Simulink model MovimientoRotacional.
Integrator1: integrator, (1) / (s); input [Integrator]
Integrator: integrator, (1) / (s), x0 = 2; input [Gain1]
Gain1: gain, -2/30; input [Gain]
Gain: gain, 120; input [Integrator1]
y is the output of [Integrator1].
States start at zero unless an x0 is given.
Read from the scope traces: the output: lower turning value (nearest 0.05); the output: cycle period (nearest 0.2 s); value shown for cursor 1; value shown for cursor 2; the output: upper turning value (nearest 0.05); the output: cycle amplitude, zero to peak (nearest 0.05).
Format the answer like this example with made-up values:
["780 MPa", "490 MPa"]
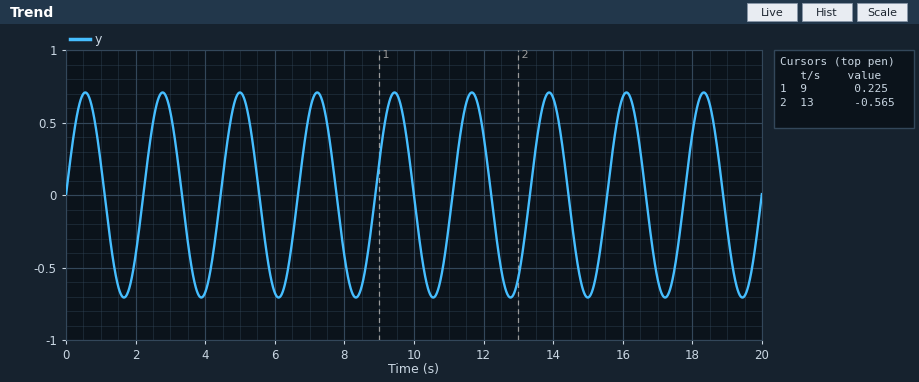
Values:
["-0.70", "2.2 s", "0.225", "-0.565", "0.70", "0.70"]
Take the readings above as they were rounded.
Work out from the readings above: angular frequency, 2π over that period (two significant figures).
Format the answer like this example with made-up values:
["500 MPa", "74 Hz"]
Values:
["2.9 rad/s"]
